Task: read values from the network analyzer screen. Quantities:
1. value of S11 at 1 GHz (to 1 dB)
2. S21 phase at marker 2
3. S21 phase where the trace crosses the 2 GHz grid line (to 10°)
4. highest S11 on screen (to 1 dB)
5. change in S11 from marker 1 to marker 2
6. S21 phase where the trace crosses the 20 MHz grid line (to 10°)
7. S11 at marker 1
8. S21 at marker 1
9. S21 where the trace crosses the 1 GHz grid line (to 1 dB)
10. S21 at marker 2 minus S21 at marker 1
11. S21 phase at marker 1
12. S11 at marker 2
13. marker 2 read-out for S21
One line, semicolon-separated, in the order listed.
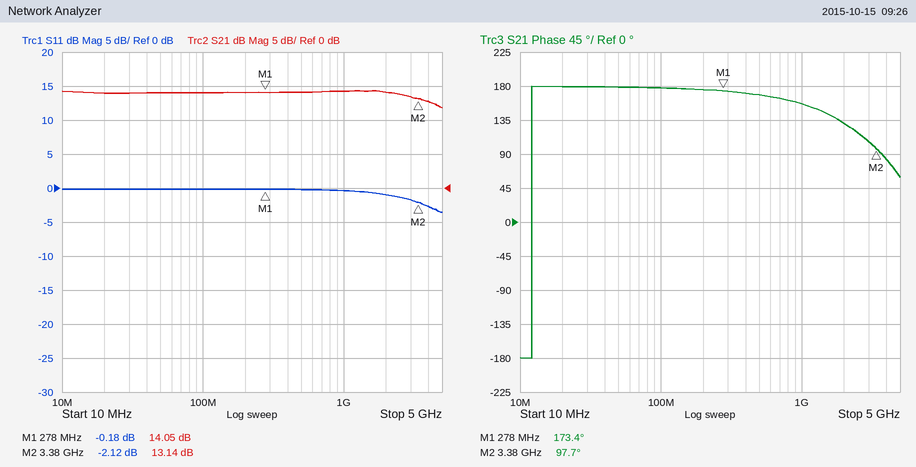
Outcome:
0 dB; 97.7°; 130°; 0 dB; -1.94 dB; 180°; -0.18 dB; 14.05 dB; 14 dB; -0.91 dB; 173.4°; -2.12 dB; 13.14 dB
